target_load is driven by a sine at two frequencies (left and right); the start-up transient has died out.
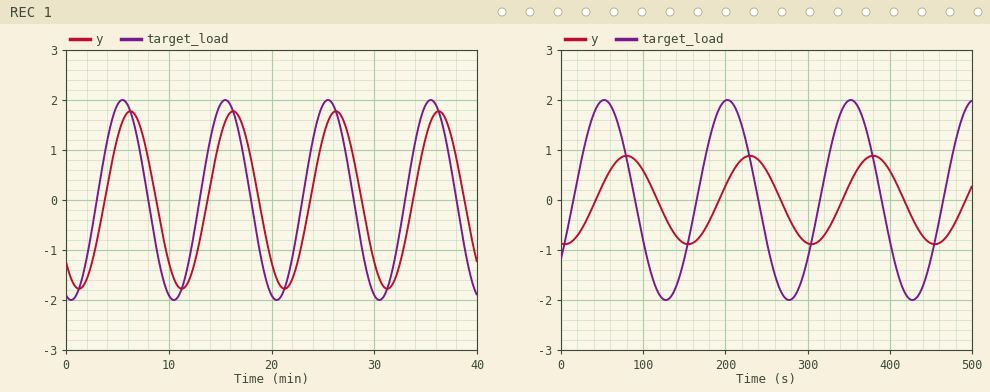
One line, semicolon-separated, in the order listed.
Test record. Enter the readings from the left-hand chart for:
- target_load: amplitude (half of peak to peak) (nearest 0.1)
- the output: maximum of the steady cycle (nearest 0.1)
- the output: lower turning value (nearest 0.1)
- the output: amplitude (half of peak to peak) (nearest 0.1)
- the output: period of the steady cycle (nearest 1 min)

2.0; 1.8; -1.8; 1.8; 10 min
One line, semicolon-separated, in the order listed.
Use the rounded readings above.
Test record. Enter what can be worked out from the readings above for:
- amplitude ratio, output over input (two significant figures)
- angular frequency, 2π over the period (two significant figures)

0.90; 0.63 rad/min
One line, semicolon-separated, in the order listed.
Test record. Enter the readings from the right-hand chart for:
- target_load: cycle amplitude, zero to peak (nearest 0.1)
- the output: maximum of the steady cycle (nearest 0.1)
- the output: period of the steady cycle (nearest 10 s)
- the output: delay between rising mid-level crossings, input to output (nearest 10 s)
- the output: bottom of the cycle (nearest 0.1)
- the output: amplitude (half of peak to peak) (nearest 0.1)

2.0; 0.9; 150 s; 30 s; -0.9; 0.9
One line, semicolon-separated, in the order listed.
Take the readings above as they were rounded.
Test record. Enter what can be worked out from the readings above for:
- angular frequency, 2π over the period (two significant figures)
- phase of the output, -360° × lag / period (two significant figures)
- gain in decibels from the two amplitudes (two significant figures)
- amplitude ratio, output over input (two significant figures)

0.042 rad/s; -72°; -6.9 dB; 0.45
